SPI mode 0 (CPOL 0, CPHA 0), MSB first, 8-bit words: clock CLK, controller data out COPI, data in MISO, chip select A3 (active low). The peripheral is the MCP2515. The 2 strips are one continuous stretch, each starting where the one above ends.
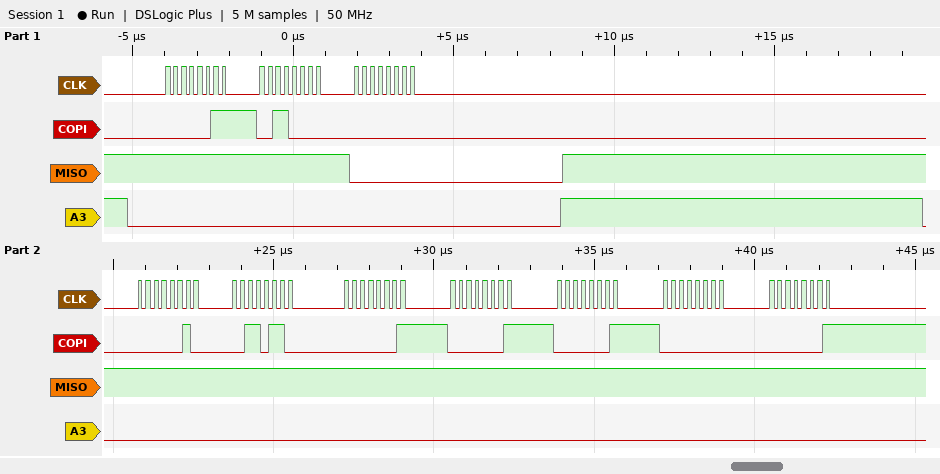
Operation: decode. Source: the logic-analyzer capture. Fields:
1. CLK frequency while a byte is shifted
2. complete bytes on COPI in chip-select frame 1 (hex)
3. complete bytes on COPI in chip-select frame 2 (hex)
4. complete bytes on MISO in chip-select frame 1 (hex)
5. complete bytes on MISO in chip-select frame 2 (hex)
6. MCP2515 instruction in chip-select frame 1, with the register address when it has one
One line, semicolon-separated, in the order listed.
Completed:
4 MHz; 03 30 00; 02 36 01 01 01 00 01; FF FF 00; FF FF FF FF FF FF FF; READ 0x30
